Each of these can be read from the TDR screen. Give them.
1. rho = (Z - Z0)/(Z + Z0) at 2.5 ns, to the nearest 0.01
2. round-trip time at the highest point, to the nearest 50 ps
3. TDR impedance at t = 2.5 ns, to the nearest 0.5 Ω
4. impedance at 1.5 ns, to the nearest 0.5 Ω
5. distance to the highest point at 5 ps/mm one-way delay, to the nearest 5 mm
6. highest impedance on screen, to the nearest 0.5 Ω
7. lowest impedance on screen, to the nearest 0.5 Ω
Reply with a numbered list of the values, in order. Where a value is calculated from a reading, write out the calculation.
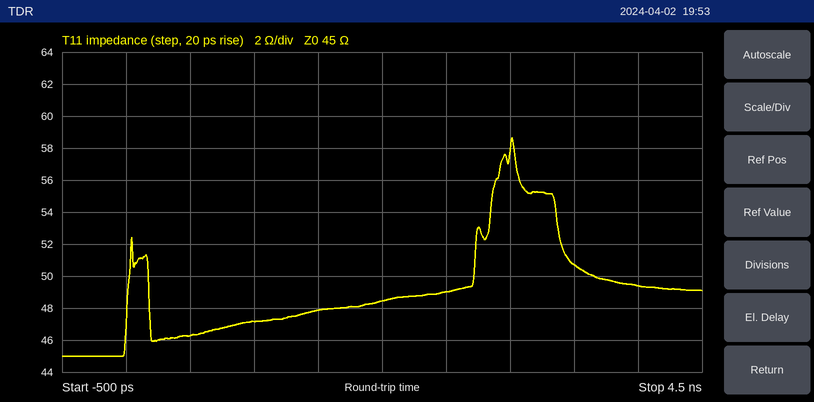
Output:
1. (49 − 45)/(49 + 45) ≈ +0.04
2. 3.00 ns
3. 49.0 Ω
4. 48.0 Ω
5. 3.00 ns / 2 / 5 ps/mm ≈ 300 mm
6. 58.5 Ω
7. 45.0 Ω
